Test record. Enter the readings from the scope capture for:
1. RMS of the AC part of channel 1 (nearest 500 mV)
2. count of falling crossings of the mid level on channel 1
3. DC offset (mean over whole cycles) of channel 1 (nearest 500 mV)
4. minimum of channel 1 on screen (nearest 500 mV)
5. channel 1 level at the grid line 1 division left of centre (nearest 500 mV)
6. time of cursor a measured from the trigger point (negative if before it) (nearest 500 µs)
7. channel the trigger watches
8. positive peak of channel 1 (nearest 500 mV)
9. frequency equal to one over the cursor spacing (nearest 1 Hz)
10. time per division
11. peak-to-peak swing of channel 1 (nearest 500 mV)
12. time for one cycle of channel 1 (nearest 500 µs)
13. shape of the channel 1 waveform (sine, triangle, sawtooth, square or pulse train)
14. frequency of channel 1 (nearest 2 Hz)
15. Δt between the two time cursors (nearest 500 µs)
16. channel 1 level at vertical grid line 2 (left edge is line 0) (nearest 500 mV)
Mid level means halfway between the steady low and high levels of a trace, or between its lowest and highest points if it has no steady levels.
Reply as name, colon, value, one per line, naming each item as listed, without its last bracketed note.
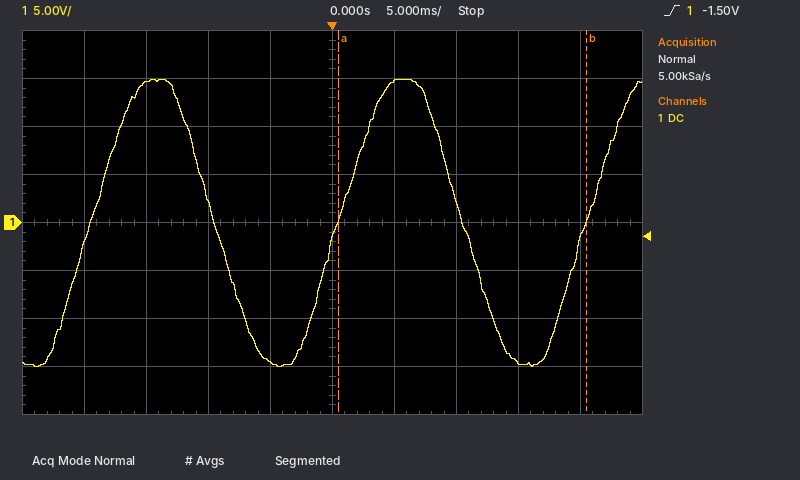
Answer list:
RMS of the AC part of channel 1: 10.5 V
count of falling crossings of the mid level on channel 1: 2
DC offset (mean over whole cycles) of channel 1: 0.0 V
minimum of channel 1 on screen: -15.0 V
channel 1 level at the grid line 1 division left of centre: -14.5 V
time of cursor a measured from the trigger point (negative if before it): +500 µs
channel the trigger watches: channel 1
positive peak of channel 1: 15.0 V
frequency equal to one over the cursor spacing: 50 Hz
time per division: 5 ms
peak-to-peak swing of channel 1: 30.0 V
time for one cycle of channel 1: 20.0 ms
shape of the channel 1 waveform: sine
frequency of channel 1: 50 Hz
Δt between the two time cursors: 20.0 ms
channel 1 level at vertical grid line 2 (left edge is line 0): 14.5 V
